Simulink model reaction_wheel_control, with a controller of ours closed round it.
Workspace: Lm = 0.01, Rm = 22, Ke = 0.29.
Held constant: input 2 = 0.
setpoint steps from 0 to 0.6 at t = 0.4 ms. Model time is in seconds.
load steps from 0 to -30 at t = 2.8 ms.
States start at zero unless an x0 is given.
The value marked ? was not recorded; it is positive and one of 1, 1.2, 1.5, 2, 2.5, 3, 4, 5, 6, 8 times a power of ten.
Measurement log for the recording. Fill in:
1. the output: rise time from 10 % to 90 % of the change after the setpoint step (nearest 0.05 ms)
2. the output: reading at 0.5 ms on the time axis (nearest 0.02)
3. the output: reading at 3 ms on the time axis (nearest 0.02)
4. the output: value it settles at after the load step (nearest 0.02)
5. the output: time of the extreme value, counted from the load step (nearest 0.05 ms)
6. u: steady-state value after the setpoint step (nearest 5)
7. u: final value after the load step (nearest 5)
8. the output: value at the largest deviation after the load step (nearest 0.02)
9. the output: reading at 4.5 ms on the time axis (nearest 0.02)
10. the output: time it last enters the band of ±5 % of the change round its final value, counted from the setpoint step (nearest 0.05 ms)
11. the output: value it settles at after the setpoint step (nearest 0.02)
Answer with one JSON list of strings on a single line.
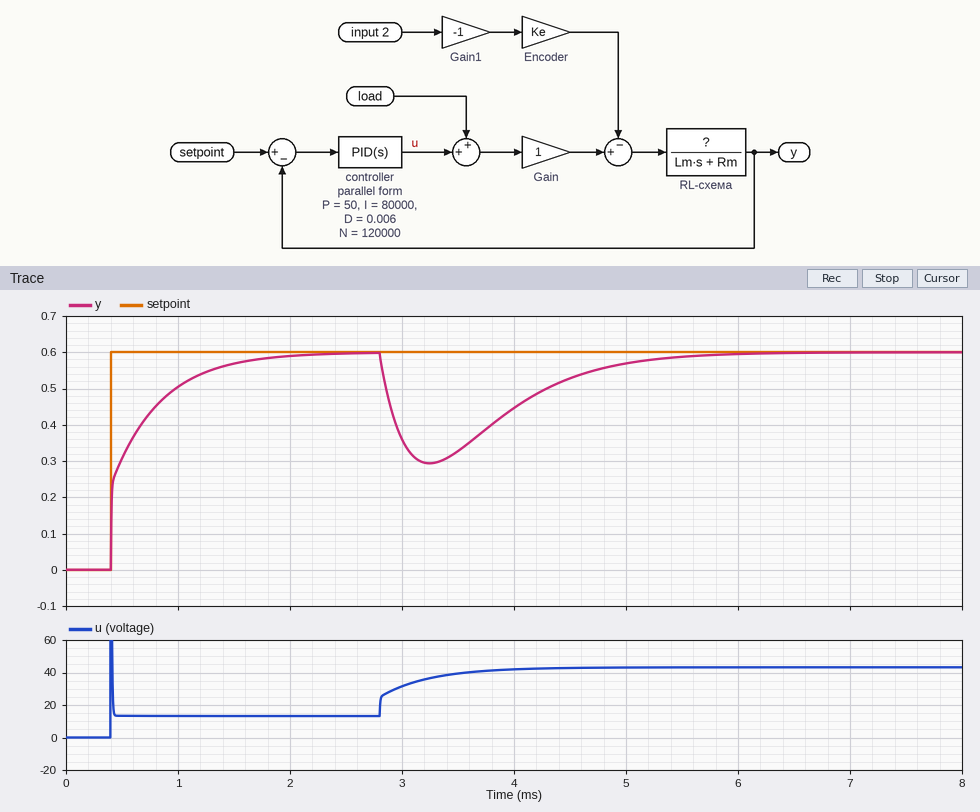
["0.80 ms", "0.30", "0.36", "0.60", "0.45 ms", "15", "45", "0.30", "0.52", "1.10 ms", "0.60"]
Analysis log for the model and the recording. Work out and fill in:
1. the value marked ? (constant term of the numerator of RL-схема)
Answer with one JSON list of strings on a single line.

["1"]
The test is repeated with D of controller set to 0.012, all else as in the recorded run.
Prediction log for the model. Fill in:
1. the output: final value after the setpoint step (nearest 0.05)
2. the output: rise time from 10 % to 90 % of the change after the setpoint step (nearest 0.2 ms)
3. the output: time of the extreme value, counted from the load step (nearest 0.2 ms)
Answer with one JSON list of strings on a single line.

["0.60", "1.0 ms", "0.6 ms"]
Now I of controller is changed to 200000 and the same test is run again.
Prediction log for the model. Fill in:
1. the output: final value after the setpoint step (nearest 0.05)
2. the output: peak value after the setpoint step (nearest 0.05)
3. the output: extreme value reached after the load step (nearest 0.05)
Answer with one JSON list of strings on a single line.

["0.60", "0.65", "0.35"]
